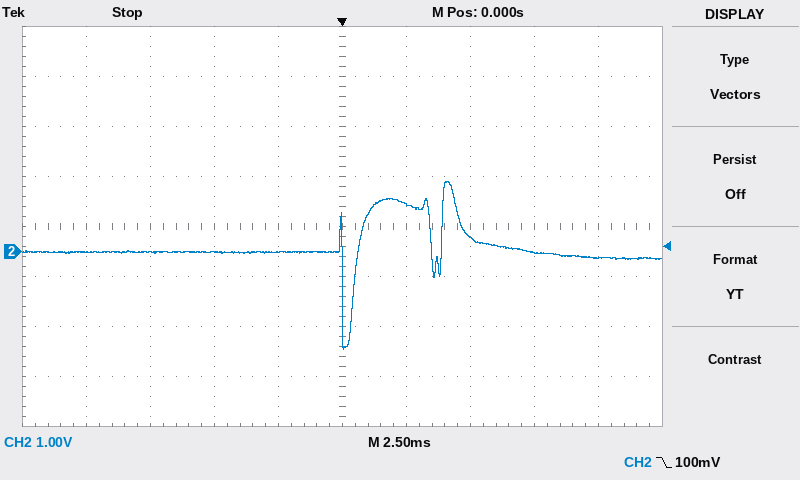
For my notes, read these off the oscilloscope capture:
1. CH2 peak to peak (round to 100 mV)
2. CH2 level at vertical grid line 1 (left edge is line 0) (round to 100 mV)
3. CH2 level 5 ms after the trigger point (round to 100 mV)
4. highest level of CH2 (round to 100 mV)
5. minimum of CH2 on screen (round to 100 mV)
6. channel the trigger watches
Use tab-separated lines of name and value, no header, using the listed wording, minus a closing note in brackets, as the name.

CH2 peak to peak	3.4 V
CH2 level at vertical grid line 1 (left edge is line 0)	0.0 V
CH2 level 5 ms after the trigger point	300 mV
highest level of CH2	1.4 V
minimum of CH2 on screen	-2.0 V
channel the trigger watches	CH2
